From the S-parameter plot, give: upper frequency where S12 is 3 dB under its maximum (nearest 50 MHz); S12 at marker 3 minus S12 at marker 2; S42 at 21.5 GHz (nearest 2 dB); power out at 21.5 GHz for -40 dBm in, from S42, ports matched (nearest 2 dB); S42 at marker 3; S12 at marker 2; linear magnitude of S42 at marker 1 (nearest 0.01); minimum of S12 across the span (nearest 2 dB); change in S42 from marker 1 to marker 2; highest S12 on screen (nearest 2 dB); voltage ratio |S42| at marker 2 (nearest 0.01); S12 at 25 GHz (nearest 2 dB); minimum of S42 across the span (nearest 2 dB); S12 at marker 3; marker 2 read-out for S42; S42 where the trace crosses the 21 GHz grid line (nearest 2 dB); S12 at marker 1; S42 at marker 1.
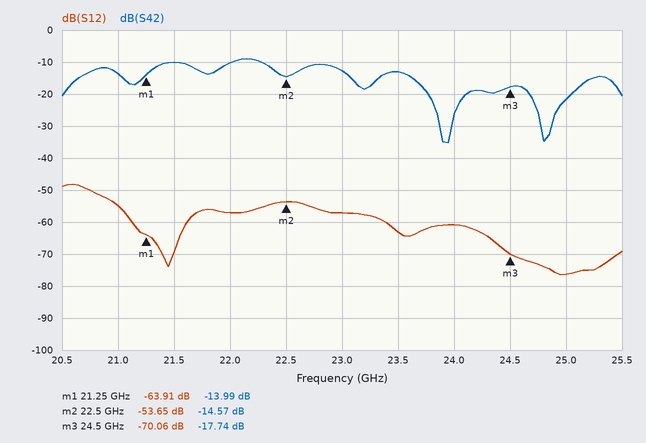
20.80 GHz
-16.41 dB
-10 dB
-50 dBm
-17.74 dB
-53.65 dB
0.20
-76 dB
-0.58 dB
-48 dB
0.19
-76 dB
-36 dB
-70.06 dB
-14.57 dB
-14 dB
-63.91 dB
-13.99 dB
